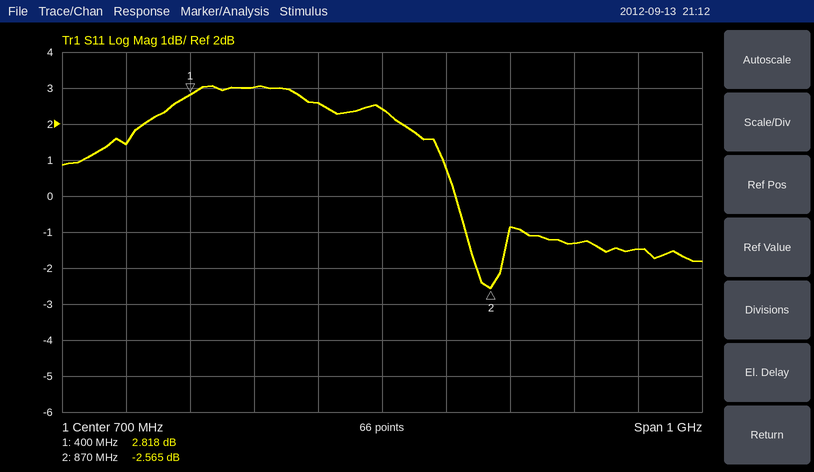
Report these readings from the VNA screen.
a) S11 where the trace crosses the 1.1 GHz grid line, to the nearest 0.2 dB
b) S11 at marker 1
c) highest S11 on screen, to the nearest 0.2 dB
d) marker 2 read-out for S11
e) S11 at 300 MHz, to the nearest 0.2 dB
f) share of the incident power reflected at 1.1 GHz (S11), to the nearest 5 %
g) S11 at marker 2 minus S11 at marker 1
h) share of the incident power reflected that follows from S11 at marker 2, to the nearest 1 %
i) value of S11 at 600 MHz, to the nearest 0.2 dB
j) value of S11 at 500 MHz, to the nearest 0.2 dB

-1.4 dB
2.818 dB
3.0 dB
-2.565 dB
1.4 dB
70 %
-5.383 dB
55 %
2.6 dB
3.0 dB
